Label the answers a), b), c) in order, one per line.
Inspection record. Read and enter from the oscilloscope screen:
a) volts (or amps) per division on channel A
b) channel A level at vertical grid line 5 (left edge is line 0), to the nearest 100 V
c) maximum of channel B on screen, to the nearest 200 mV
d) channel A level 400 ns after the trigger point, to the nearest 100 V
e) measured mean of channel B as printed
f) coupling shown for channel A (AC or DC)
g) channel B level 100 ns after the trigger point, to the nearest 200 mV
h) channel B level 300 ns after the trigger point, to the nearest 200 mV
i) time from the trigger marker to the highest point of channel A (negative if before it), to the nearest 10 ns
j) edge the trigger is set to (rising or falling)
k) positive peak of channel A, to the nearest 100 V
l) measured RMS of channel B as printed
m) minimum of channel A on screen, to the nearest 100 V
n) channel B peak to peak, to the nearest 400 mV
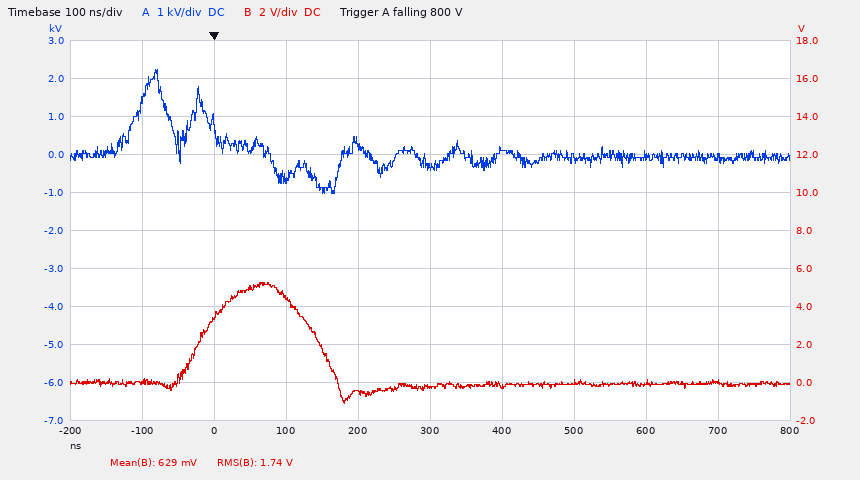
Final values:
a) 1 kV
b) -300 V
c) 5.2 V
d) 100 V
e) 629 mV
f) DC
g) 4.4 V
h) -200 mV
i) -80 ns
j) falling
k) 2.2 kV
l) 1.74 V
m) -1.0 kV
n) 6.4 V
